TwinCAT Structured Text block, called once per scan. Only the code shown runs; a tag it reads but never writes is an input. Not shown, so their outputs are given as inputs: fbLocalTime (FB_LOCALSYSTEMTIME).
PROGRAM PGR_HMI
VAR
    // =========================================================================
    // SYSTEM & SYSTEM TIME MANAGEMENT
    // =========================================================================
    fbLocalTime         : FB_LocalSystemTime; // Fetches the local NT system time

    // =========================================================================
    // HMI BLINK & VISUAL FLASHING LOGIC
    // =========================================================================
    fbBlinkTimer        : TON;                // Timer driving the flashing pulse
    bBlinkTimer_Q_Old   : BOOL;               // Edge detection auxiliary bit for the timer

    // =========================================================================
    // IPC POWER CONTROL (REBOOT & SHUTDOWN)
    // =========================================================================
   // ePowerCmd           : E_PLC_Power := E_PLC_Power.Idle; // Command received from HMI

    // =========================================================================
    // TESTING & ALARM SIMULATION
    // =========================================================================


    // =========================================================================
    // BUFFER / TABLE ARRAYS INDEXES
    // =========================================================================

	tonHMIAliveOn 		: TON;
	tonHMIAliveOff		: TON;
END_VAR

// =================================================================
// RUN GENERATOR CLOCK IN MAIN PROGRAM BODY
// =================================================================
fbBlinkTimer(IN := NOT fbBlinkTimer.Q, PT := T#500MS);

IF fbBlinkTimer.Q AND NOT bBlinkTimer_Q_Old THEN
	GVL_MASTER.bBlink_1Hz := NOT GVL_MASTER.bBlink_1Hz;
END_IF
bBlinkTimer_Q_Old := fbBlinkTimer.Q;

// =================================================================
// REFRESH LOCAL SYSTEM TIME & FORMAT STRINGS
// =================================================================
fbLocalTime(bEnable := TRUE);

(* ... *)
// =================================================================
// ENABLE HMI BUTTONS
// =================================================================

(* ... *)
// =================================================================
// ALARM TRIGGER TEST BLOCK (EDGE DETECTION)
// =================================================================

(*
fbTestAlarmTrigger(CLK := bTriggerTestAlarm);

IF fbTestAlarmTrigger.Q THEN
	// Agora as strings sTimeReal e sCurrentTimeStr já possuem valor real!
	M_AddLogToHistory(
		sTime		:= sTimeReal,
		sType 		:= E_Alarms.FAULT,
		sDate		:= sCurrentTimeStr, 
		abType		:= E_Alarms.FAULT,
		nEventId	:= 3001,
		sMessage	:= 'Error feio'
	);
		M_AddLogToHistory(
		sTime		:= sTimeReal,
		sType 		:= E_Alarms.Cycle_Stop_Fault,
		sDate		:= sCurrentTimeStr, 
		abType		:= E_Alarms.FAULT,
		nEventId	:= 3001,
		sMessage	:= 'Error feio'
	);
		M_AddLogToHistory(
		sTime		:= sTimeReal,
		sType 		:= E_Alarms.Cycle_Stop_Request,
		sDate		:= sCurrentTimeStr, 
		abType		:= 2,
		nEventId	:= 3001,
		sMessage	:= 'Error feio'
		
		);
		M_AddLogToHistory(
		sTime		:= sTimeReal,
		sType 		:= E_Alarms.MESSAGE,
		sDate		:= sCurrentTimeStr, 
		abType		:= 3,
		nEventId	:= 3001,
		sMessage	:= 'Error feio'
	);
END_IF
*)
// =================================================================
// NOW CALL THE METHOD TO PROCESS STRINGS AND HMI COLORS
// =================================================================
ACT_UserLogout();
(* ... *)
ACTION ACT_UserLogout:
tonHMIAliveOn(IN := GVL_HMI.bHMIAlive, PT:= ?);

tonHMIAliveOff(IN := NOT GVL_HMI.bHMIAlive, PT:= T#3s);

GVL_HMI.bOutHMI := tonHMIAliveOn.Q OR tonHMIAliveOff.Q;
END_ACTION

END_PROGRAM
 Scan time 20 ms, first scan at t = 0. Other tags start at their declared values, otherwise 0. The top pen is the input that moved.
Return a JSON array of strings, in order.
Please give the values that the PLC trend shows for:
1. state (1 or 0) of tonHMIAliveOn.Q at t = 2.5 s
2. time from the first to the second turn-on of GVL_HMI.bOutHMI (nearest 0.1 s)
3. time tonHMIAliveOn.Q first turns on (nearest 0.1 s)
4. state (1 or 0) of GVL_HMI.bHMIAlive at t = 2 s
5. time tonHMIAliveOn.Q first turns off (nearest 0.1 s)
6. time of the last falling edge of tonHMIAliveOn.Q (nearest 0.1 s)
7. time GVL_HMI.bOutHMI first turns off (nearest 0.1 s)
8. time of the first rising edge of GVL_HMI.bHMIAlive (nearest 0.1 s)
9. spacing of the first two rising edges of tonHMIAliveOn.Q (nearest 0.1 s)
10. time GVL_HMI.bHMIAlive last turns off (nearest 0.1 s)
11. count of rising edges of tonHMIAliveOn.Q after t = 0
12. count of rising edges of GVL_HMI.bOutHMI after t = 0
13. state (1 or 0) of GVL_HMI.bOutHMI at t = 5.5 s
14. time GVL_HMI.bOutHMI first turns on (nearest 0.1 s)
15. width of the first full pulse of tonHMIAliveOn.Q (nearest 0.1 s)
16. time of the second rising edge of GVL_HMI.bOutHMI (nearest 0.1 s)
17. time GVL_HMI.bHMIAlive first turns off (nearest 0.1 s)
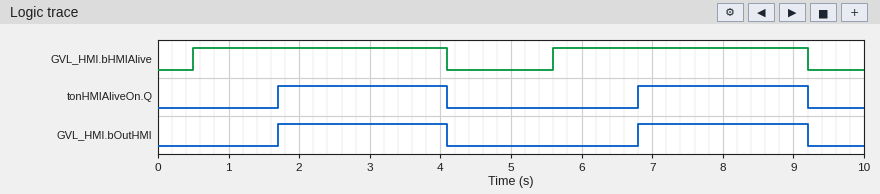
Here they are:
["1", "5.1 s", "1.7 s", "1", "4.1 s", "9.2 s", "4.1 s", "0.5 s", "5.1 s", "9.2 s", "2", "2", "0", "1.7 s", "2.4 s", "6.8 s", "4.1 s"]
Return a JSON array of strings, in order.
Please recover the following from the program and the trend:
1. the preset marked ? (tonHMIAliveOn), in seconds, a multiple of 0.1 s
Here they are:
["1.2 s"]
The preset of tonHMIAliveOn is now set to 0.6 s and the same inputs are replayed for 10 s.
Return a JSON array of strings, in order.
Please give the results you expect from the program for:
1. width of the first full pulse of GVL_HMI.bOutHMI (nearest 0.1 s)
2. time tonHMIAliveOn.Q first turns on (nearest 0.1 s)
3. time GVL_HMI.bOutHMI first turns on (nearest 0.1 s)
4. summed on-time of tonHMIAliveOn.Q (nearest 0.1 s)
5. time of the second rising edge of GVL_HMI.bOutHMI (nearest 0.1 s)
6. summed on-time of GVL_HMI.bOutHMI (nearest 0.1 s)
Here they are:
["3.0 s", "1.1 s", "1.1 s", "6.0 s", "6.2 s", "6.0 s"]
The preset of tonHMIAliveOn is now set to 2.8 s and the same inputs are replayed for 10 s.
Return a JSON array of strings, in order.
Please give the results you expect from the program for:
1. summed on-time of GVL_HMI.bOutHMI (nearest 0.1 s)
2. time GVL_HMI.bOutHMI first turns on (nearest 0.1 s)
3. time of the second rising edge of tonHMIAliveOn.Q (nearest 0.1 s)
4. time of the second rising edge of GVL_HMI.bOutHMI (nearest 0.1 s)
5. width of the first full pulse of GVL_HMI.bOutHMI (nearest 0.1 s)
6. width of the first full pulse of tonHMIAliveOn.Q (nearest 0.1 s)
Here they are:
["1.6 s", "3.3 s", "8.4 s", "8.4 s", "0.8 s", "0.8 s"]
